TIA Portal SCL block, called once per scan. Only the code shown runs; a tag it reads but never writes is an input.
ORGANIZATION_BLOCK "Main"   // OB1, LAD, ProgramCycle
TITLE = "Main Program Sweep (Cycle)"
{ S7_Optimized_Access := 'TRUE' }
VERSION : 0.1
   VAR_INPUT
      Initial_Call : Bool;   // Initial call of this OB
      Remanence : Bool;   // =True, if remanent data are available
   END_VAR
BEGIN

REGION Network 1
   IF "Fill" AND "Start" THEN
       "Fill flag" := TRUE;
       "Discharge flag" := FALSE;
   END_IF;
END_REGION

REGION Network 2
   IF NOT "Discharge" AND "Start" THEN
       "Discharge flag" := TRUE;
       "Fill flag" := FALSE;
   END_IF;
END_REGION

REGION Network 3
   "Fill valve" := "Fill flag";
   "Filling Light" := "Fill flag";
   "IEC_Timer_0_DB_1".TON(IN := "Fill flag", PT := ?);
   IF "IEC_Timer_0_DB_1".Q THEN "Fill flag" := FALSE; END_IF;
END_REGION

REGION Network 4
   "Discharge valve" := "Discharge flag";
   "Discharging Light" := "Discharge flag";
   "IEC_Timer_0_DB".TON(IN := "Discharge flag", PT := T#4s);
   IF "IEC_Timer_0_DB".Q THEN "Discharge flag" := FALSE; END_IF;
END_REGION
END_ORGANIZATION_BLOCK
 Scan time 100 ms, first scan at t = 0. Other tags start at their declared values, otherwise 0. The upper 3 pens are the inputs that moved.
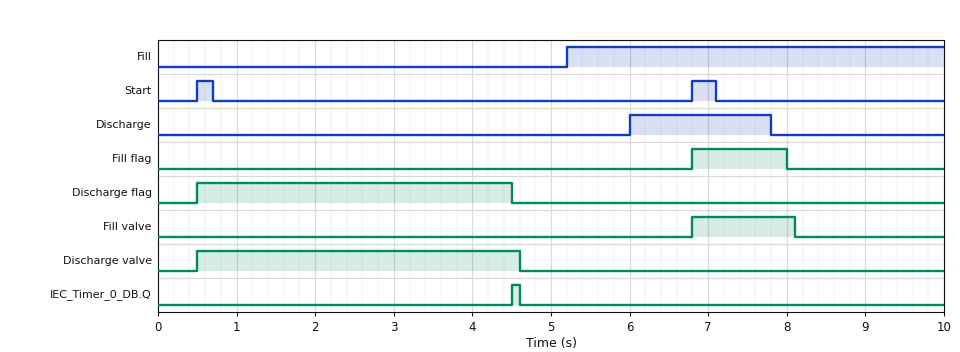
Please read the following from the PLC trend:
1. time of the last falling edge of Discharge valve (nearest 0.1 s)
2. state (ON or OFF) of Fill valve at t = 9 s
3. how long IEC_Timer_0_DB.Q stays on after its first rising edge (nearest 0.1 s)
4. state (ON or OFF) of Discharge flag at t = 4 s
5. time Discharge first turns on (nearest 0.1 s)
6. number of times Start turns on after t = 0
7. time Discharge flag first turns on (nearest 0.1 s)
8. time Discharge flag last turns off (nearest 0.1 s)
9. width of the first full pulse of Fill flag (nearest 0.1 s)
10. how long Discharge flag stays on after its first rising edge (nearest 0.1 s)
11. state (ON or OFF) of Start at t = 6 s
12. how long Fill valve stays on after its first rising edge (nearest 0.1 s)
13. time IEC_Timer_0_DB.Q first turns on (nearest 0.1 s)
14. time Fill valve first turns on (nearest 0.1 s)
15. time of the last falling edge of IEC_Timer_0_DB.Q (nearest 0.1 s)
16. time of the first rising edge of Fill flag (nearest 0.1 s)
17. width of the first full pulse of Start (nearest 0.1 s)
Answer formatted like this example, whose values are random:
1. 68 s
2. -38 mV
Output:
1. 4.6 s
2. OFF
3. 0.1 s
4. ON
5. 6.0 s
6. 2
7. 0.5 s
8. 4.5 s
9. 1.2 s
10. 4.0 s
11. OFF
12. 1.3 s
13. 4.5 s
14. 6.8 s
15. 4.6 s
16. 6.8 s
17. 0.2 s
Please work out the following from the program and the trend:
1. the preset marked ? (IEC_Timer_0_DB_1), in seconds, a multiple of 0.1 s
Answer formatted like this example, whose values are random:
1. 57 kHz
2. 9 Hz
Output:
1. 1.2 s
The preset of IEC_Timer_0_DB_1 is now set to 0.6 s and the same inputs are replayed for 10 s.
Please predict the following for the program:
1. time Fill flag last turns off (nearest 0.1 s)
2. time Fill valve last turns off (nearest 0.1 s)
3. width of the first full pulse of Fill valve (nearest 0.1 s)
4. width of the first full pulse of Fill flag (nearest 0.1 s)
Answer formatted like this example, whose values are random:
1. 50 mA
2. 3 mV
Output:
1. 7.4 s
2. 7.5 s
3. 0.7 s
4. 0.6 s
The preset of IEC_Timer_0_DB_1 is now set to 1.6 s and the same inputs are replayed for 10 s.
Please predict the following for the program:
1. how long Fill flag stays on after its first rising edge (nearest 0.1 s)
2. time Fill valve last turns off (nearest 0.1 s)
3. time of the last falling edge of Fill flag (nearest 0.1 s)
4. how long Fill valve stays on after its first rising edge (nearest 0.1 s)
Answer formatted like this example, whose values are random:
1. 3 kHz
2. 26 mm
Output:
1. 1.6 s
2. 8.5 s
3. 8.4 s
4. 1.7 s
